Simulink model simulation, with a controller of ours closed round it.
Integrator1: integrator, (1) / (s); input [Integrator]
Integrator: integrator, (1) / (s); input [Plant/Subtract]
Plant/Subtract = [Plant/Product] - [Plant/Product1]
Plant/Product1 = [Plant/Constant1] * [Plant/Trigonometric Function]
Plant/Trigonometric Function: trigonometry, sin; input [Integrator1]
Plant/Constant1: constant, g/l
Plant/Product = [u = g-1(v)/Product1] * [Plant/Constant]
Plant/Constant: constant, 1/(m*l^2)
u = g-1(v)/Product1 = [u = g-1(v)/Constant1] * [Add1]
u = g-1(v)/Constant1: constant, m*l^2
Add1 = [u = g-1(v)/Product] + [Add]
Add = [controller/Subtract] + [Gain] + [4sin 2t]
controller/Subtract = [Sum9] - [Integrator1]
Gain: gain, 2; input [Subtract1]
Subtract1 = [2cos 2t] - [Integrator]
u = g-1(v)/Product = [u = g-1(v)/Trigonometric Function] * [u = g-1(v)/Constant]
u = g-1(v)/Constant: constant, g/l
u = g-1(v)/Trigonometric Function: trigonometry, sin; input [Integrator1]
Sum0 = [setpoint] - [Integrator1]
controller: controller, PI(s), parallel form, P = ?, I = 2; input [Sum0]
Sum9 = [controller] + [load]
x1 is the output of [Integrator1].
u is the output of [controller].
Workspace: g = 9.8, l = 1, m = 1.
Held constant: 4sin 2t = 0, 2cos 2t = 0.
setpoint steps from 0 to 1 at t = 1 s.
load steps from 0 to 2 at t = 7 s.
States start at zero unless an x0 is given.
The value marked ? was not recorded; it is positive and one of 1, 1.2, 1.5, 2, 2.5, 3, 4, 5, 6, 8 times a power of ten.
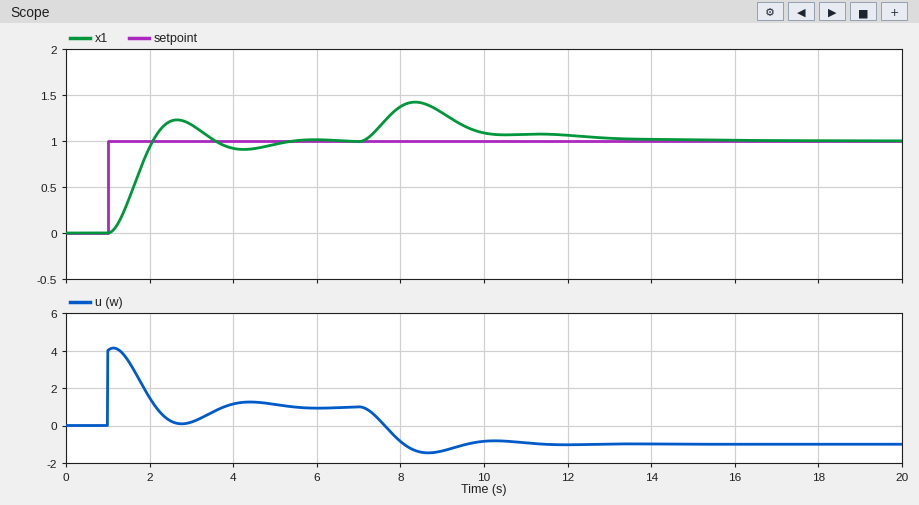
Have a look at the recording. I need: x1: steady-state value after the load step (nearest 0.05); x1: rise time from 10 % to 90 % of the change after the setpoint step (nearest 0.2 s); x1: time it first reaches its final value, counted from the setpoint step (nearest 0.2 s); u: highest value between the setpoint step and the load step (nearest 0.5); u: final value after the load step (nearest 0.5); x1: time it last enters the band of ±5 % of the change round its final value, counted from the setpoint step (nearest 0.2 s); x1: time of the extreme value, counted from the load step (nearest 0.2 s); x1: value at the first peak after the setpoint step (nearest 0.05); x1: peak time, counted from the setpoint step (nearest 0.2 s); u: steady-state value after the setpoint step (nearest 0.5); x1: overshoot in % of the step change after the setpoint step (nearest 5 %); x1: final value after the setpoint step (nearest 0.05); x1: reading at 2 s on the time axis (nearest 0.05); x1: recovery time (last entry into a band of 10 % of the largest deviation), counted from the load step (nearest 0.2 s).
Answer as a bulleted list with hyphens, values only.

- 1.00
- 0.8 s
- 1.0 s
- 4.0
- -1.0
- 3.8 s
- 1.4 s
- 1.25
- 1.6 s
- 1.0
- 25 %
- 1.00
- 0.95
- 5.6 s
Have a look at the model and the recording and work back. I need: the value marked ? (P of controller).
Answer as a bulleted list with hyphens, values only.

- 4
